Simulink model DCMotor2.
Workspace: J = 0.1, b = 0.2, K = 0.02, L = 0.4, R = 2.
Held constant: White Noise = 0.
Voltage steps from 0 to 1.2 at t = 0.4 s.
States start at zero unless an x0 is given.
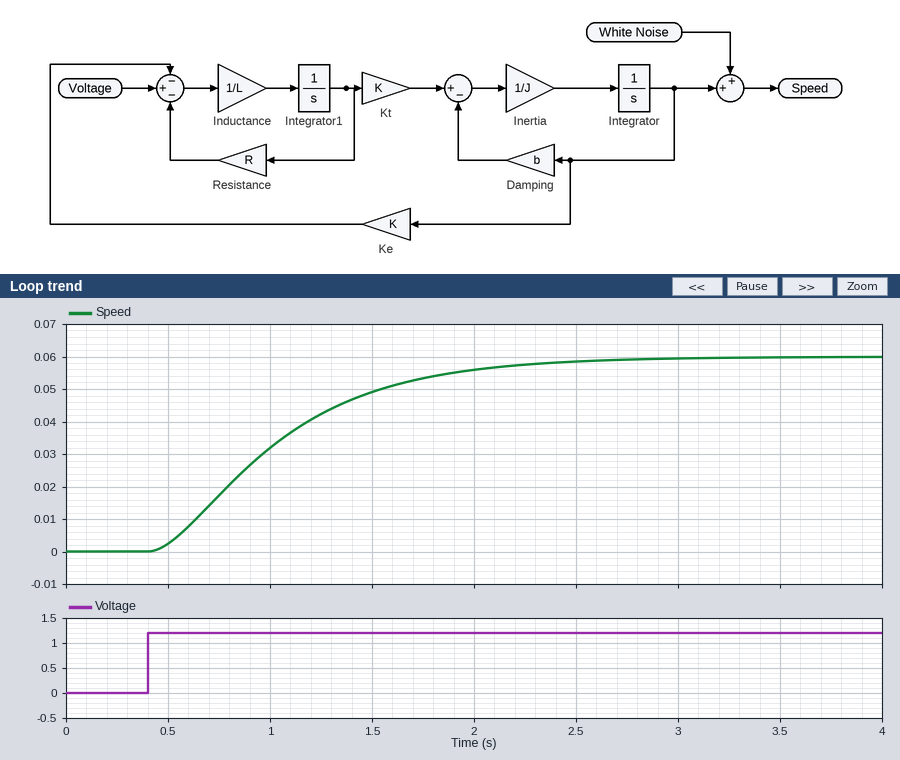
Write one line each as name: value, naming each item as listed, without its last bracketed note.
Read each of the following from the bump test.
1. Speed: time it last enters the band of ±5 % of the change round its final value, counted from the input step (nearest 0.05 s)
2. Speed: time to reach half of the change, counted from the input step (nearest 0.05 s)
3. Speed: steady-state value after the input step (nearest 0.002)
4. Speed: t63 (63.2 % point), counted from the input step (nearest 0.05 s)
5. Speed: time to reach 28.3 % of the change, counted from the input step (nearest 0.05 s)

Speed: time it last enters the band of ±5 % of the change round its final value, counted from the input step: 1.75 s
Speed: time to reach half of the change, counted from the input step: 0.55 s
Speed: steady-state value after the input step: 0.060
Speed: t63 (63.2 % point), counted from the input step: 0.75 s
Speed: time to reach 28.3 % of the change, counted from the input step: 0.35 s
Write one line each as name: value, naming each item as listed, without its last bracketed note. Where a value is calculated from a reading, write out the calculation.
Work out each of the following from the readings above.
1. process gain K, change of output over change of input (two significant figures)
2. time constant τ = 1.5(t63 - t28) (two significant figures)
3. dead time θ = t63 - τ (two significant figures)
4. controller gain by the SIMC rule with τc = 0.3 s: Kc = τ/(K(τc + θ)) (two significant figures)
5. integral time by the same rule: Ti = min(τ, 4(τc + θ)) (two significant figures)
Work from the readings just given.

process gain K, change of output over change of input: (0.06 - 0) / 1.2 = 0.050
time constant τ = 1.5(t63 - t28): 1.5 × (0.75 - 0.35) = 0.60 s
dead time θ = t63 - τ: 0.75 - 0.6 = 0.15 s
controller gain by the SIMC rule with τc = 0.3 s: Kc = τ/(K(τc + θ)): 0.6 / (0.05 × (0.3 + 0.15)) = 27
integral time by the same rule: Ti = min(τ, 4(τc + θ)): min(0.6, 4 × (0.3 + 0.15)) = 0.60 s
